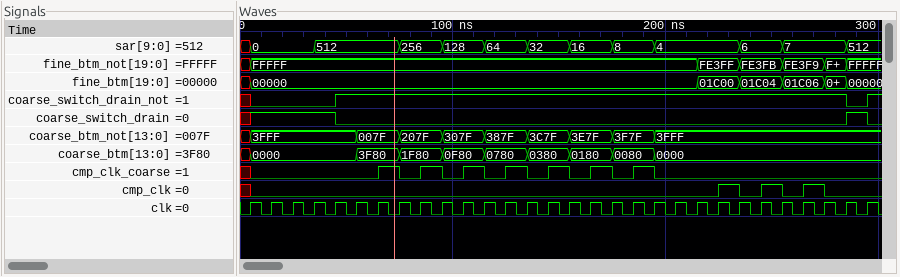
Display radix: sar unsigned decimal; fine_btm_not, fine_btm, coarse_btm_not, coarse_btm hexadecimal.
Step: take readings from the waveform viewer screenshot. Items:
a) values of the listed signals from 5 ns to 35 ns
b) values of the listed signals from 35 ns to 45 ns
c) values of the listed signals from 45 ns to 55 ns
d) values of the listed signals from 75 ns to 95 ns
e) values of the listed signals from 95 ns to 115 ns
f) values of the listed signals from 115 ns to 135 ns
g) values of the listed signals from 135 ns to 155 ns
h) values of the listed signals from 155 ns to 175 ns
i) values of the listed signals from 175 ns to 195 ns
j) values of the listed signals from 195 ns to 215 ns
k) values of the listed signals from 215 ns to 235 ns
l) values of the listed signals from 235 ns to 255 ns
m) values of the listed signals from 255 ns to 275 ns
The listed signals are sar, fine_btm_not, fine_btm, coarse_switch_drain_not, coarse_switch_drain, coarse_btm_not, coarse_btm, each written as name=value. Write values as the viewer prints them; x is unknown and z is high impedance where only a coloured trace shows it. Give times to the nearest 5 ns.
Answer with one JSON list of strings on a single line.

["sar=0, fine_btm_not=FFFFF, fine_btm=00000, coarse_switch_drain_not=0, coarse_switch_drain=1, coarse_btm_not=3FFF, coarse_btm=0000", "sar=512, fine_btm_not=FFFFF, fine_btm=00000, coarse_switch_drain_not=0, coarse_switch_drain=1, coarse_btm_not=3FFF, coarse_btm=0000", "sar=512, fine_btm_not=FFFFF, fine_btm=00000, coarse_switch_drain_not=1, coarse_switch_drain=0, coarse_btm_not=3FFF, coarse_btm=0000", "sar=256, fine_btm_not=FFFFF, fine_btm=00000, coarse_switch_drain_not=1, coarse_switch_drain=0, coarse_btm_not=207F, coarse_btm=1F80", "sar=128, fine_btm_not=FFFFF, fine_btm=00000, coarse_switch_drain_not=1, coarse_switch_drain=0, coarse_btm_not=307F, coarse_btm=0F80", "sar=64, fine_btm_not=FFFFF, fine_btm=00000, coarse_switch_drain_not=1, coarse_switch_drain=0, coarse_btm_not=387F, coarse_btm=0780", "sar=32, fine_btm_not=FFFFF, fine_btm=00000, coarse_switch_drain_not=1, coarse_switch_drain=0, coarse_btm_not=3C7F, coarse_btm=0380", "sar=16, fine_btm_not=FFFFF, fine_btm=00000, coarse_switch_drain_not=1, coarse_switch_drain=0, coarse_btm_not=3E7F, coarse_btm=0180", "sar=8, fine_btm_not=FFFFF, fine_btm=00000, coarse_switch_drain_not=1, coarse_switch_drain=0, coarse_btm_not=3F7F, coarse_btm=0080", "sar=4, fine_btm_not=FFFFF, fine_btm=00000, coarse_switch_drain_not=1, coarse_switch_drain=0, coarse_btm_not=3FFF, coarse_btm=0000", "sar=4, fine_btm_not=FE3FF, fine_btm=01C00, coarse_switch_drain_not=1, coarse_switch_drain=0, coarse_btm_not=3FFF, coarse_btm=0000", "sar=6, fine_btm_not=FE3FB, fine_btm=01C04, coarse_switch_drain_not=1, coarse_switch_drain=0, coarse_btm_not=3FFF, coarse_btm=0000", "sar=7, fine_btm_not=FE3F9, fine_btm=01C06, coarse_switch_drain_not=1, coarse_switch_drain=0, coarse_btm_not=3FFF, coarse_btm=0000"]
